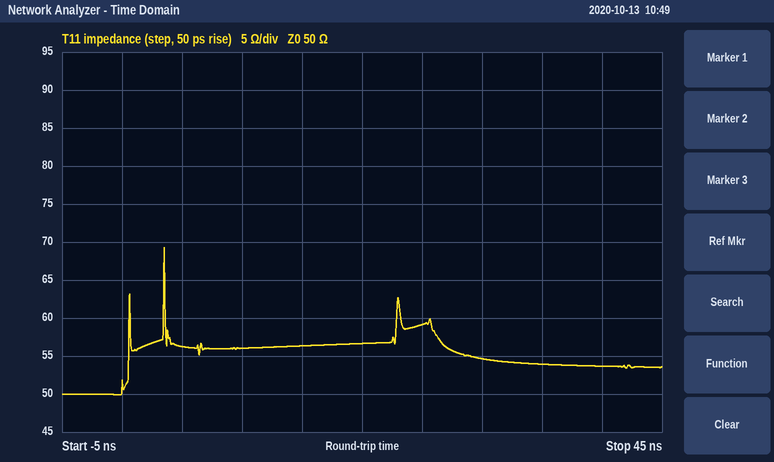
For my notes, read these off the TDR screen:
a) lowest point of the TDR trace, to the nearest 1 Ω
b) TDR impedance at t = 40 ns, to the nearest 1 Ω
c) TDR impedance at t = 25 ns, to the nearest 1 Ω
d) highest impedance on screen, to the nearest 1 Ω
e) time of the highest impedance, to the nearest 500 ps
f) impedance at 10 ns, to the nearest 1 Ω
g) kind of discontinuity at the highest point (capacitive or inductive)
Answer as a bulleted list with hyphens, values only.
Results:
- 50 Ω
- 54 Ω
- 59 Ω
- 69 Ω
- 3.5 ns
- 56 Ω
- inductive
